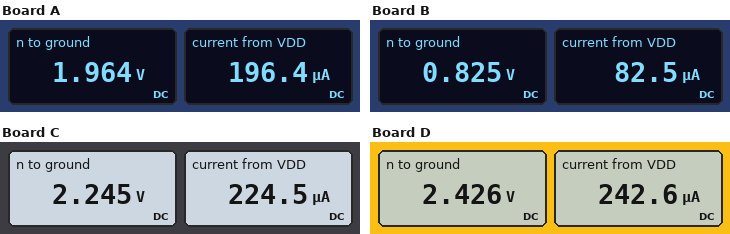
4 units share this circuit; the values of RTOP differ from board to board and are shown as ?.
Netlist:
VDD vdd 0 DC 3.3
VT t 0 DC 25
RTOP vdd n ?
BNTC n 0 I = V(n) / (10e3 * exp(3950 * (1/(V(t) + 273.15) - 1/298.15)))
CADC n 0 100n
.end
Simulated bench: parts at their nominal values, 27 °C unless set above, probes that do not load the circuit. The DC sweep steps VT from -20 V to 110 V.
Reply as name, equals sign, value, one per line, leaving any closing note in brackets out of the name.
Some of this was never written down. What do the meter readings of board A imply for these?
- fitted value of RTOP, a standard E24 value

fitted value of RTOP, a standard E24 value = 6.8 kΩ
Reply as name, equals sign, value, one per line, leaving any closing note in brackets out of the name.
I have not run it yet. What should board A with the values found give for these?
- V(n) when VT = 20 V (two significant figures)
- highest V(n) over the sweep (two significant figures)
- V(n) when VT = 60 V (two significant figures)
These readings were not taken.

V(n) when VT = 20 V = 2.1 V
highest V(n) over the sweep = 3.1 V
V(n) when VT = 60 V = 880 mV
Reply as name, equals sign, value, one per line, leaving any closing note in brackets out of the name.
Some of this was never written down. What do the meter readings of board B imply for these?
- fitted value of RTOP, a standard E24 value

fitted value of RTOP, a standard E24 value = 30 kΩ
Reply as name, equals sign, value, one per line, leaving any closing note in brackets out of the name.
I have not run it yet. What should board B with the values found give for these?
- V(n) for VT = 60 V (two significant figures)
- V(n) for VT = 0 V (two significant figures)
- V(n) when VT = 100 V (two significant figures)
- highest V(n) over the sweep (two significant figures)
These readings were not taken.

V(n) for VT = 60 V = 250 mV
V(n) for VT = 0 V = 1.7 V
V(n) when VT = 100 V = 75 mV
highest V(n) over the sweep = 2.6 V
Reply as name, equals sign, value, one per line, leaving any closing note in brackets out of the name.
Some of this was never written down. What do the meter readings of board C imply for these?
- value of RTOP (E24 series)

value of RTOP = 4.7 kΩ
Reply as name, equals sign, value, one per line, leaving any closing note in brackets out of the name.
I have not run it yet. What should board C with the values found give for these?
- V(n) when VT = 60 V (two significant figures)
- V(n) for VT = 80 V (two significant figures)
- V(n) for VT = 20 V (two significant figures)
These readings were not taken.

V(n) when VT = 60 V = 1.1 V
V(n) for VT = 80 V = 700 mV
V(n) for VT = 20 V = 2.4 V
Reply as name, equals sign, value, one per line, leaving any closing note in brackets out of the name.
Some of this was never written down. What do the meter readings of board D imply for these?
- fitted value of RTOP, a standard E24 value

fitted value of RTOP, a standard E24 value = 3.6 kΩ
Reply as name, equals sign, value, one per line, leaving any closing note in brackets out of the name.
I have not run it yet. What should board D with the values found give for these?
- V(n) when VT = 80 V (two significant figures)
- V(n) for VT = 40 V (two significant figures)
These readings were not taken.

V(n) when VT = 80 V = 860 mV
V(n) for VT = 40 V = 2.0 V
